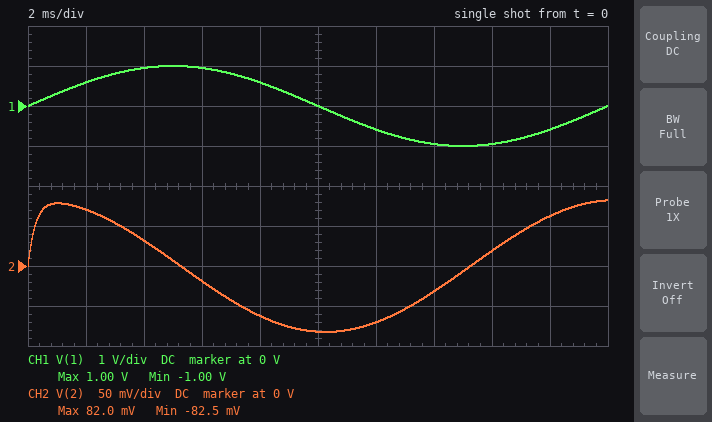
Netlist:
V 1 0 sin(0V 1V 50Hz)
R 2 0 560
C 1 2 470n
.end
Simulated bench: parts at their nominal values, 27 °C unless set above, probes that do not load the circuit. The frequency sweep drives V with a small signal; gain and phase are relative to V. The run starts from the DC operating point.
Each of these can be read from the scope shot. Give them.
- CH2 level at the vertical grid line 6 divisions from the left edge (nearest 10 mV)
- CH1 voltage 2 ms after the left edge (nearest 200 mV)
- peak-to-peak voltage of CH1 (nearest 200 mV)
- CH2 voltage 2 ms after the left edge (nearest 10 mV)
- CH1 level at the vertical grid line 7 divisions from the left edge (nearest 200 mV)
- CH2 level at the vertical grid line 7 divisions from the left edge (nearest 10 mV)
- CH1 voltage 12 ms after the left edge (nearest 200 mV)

-70 mV
600 mV
2.0 V
70 mV
-1.0 V
-30 mV
-600 mV
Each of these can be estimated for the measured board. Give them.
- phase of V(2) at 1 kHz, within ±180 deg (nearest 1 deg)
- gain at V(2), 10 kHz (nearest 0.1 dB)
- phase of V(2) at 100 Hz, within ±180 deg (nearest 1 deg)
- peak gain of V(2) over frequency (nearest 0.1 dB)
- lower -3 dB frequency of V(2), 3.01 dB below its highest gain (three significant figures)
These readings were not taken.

31 deg
0 dB
81 deg
0 dB
605 Hz
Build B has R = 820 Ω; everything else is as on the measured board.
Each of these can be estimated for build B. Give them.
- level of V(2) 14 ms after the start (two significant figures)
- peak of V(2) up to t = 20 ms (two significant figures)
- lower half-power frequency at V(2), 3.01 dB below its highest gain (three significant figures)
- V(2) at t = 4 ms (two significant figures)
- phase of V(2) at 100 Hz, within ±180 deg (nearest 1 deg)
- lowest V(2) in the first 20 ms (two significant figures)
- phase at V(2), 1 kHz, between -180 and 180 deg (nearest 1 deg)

-51 mV
120 mV
413 Hz
51 mV
76 deg
-120 mV
22 deg
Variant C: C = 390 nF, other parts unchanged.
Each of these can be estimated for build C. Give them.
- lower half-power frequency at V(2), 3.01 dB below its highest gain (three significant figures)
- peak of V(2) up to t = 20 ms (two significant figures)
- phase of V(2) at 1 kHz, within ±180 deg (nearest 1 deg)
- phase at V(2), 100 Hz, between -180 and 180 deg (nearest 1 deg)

729 Hz
68 mV
36 deg
82 deg
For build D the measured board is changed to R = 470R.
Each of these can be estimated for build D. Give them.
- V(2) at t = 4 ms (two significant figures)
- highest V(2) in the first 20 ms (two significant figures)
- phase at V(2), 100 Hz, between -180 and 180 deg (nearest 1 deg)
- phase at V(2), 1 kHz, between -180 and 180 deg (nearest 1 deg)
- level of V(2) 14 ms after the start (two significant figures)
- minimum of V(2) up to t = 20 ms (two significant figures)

26 mV
69 mV
82 deg
36 deg
-26 mV
-69 mV
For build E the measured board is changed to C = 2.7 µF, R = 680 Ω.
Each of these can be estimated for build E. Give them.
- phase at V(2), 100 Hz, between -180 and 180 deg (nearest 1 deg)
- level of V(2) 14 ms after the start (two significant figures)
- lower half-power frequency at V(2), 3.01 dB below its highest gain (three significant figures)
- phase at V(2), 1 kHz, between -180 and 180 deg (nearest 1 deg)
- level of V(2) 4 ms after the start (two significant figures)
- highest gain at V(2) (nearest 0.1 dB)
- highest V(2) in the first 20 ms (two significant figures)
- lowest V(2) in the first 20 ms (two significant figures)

41 deg
-370 mV
86.7 Hz
5 deg
320 mV
0 dB
430 mV
-500 mV
